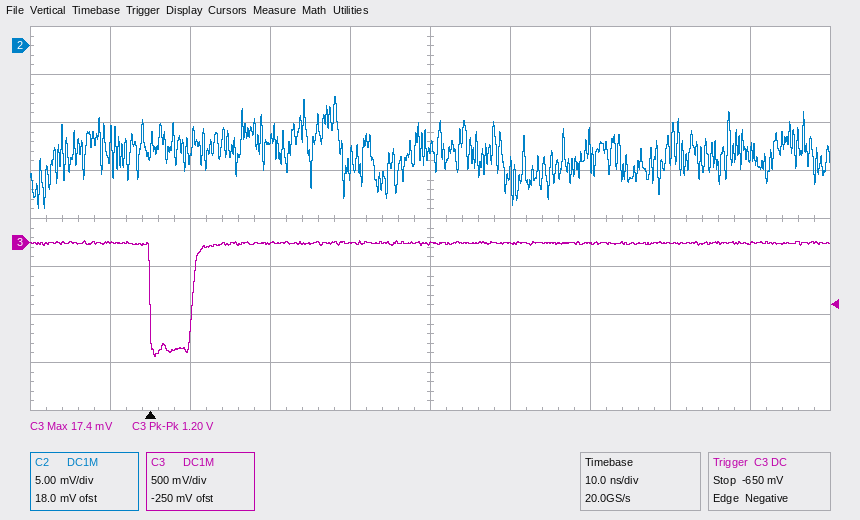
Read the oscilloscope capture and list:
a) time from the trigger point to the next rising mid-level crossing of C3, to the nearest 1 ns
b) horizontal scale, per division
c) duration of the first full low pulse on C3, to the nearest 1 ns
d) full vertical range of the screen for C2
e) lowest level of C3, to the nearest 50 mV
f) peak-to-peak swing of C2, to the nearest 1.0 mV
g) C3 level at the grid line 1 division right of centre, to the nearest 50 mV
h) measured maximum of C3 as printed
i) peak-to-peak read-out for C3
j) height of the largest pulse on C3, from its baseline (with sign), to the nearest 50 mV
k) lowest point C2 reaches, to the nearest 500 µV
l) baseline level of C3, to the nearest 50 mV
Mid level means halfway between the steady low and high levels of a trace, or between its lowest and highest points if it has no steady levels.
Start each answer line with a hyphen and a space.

- 5 ns
- 10 ns
- 5 ns
- 40 mV
- -1.20 V
- 12.0 mV
- 0 mV
- 17.4 mV
- 1.20 V
- -1.20 V
- -17.0 mV
- 0 mV
